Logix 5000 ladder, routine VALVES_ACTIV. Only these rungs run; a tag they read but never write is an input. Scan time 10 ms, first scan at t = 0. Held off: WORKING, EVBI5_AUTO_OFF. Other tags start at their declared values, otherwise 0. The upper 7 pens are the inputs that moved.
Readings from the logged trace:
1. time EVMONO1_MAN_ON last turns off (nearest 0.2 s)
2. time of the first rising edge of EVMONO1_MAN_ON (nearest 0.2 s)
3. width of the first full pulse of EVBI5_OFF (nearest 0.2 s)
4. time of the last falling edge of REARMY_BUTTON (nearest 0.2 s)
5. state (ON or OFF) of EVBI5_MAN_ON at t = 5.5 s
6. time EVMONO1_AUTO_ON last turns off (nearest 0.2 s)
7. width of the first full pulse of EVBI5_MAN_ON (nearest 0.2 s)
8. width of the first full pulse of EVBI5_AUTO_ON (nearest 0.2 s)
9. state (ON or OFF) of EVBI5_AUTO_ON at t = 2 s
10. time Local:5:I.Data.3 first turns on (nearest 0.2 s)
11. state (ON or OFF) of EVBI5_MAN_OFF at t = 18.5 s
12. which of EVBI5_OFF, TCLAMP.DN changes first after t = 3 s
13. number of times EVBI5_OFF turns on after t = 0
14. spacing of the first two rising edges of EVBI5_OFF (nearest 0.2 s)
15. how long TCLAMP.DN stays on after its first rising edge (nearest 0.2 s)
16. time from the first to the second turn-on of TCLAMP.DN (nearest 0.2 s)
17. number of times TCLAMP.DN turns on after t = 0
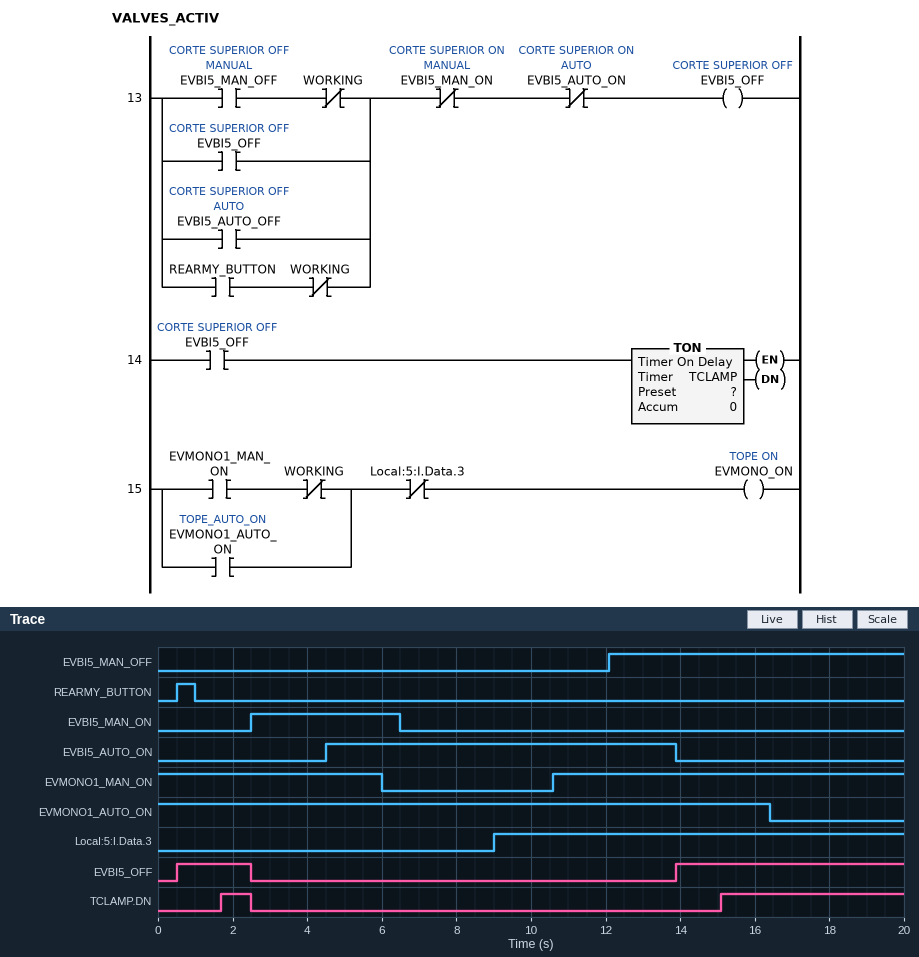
6.0 s
10.6 s
2.0 s
1.0 s
ON
16.4 s
4.0 s
9.4 s
OFF
9.0 s
ON
EVBI5_OFF
2
13.4 s
0.8 s
13.4 s
2
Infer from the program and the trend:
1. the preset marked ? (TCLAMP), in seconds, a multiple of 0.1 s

1.2 s
